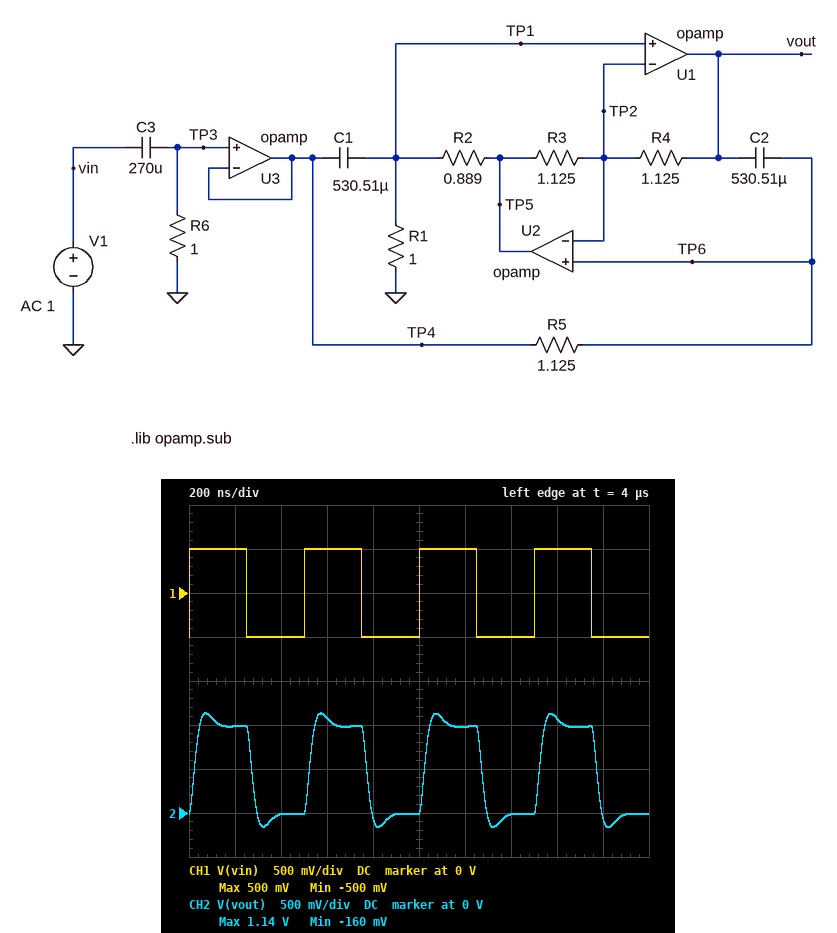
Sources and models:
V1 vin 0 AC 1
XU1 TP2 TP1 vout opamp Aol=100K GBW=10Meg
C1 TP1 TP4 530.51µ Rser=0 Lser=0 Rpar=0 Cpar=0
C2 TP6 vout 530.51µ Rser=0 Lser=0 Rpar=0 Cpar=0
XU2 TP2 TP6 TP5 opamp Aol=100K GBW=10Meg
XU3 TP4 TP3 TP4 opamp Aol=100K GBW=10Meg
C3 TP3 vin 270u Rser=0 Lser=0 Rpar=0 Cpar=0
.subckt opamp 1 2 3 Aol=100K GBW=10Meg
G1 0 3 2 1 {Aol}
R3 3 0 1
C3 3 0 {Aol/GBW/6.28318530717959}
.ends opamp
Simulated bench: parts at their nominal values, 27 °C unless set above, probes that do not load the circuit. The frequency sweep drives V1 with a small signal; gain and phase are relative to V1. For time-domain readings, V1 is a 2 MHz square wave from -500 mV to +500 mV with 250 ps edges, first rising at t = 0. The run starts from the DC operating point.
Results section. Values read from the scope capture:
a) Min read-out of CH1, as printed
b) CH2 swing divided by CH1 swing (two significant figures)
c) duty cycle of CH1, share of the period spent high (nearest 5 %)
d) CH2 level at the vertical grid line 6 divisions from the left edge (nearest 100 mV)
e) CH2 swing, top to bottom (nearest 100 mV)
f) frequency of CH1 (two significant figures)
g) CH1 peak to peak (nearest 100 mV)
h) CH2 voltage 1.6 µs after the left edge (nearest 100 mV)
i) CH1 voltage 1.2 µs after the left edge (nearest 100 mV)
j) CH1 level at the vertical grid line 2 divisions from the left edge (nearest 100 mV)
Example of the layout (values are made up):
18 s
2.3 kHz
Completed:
-500 mV
1.3
50 %
1.0 V
1.3 V
2.0 MHz
1.0 V
1.1 V
500 mV
-500 mV
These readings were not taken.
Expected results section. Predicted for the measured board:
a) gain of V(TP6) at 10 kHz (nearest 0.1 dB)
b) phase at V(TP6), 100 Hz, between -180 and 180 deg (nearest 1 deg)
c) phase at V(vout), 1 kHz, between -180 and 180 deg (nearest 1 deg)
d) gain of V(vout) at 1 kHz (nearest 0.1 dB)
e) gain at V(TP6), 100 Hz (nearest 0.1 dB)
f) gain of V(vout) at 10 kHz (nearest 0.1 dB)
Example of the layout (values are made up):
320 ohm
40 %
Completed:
0 dB
60 deg
49 deg
-1.0 dB
-16.1 dB
0 dB
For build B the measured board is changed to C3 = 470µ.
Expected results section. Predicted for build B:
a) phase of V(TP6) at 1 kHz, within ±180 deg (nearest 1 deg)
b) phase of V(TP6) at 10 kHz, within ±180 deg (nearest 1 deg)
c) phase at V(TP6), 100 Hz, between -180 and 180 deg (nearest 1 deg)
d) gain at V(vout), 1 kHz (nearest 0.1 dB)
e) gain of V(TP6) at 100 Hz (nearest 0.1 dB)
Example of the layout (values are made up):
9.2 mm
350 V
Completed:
37 deg
4 deg
53 deg
-0.2 dB
-11.5 dB
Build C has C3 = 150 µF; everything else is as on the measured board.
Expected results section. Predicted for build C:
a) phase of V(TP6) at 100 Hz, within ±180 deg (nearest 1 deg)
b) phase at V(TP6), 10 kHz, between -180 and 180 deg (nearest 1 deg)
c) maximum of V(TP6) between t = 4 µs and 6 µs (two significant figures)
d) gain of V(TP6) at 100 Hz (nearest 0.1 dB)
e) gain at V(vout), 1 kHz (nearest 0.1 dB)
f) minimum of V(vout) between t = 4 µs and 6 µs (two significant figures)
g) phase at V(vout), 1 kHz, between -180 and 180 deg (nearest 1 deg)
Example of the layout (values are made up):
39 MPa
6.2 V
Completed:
64 deg
8 deg
1.1 V
-21.1 dB
-3.0 dB
-170 mV
65 deg
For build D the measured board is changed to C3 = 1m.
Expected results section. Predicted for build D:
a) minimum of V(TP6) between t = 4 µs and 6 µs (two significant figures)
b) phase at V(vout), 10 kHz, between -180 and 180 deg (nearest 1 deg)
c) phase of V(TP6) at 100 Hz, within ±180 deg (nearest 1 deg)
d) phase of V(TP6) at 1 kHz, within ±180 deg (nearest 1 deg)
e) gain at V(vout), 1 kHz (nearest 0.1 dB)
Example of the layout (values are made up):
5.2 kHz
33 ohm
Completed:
-150 mV
3 deg
37 deg
27 deg
0.2 dB
